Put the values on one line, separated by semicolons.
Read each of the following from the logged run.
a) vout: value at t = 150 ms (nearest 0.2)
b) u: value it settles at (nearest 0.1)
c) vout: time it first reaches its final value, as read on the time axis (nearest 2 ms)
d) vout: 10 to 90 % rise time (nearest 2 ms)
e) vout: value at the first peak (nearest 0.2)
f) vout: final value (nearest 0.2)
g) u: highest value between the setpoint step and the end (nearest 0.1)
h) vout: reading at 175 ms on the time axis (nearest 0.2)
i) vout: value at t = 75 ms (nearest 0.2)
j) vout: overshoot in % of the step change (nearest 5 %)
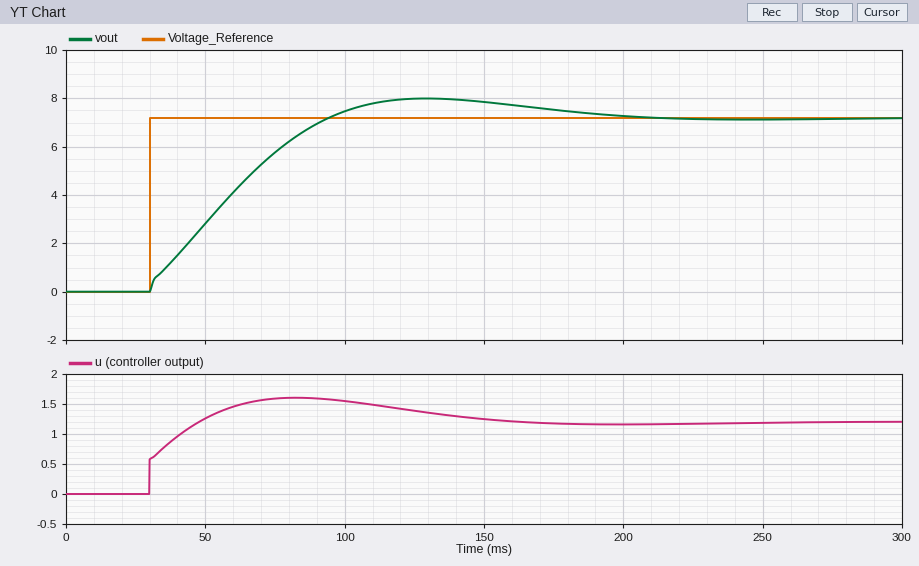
7.8; 1.2; 94 ms; 50 ms; 8.0; 7.2; 1.6; 7.6; 5.8; 10 %
